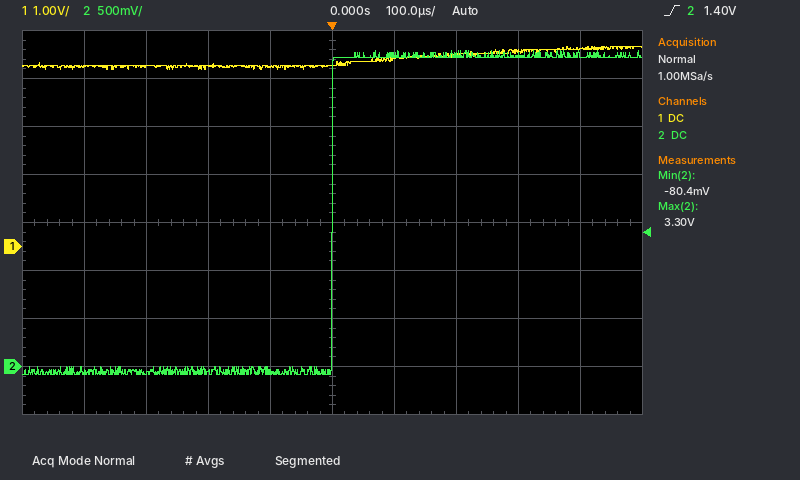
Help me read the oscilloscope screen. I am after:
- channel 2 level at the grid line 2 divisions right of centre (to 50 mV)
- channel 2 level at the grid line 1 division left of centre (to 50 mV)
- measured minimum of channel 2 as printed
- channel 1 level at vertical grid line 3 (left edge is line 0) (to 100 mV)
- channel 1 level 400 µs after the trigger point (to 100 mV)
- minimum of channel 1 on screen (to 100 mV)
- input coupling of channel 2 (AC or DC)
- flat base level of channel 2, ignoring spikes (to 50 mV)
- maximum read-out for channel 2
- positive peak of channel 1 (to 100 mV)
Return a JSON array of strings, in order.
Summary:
["3.25 V", "-50 mV", "-80.4 mV", "3.7 V", "4.1 V", "3.7 V", "DC", "-50 mV", "3.30 V", "4.2 V"]
